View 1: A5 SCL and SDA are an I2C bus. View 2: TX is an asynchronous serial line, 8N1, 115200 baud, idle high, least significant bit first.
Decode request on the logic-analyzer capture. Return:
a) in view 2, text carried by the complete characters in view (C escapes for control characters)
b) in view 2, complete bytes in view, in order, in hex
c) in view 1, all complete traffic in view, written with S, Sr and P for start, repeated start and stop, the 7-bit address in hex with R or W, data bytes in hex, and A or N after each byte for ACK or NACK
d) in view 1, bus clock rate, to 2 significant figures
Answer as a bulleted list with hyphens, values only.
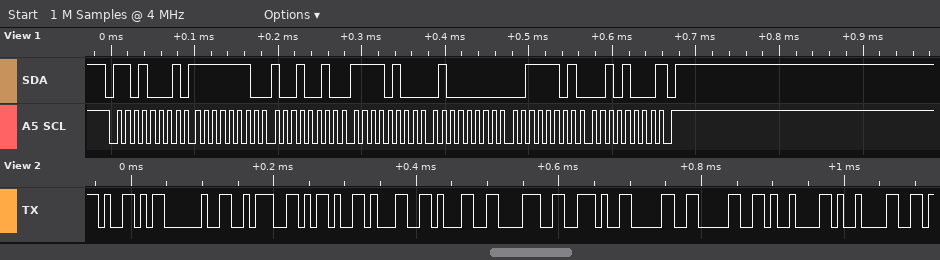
- "Y :-118.00\t\t"
- 59 20 3A 2D 31 31 38 2E 30 30 09 09
- S 68R A FE A 92 A F4 A 40 A 3D A 28 N P
- 100 kHz
